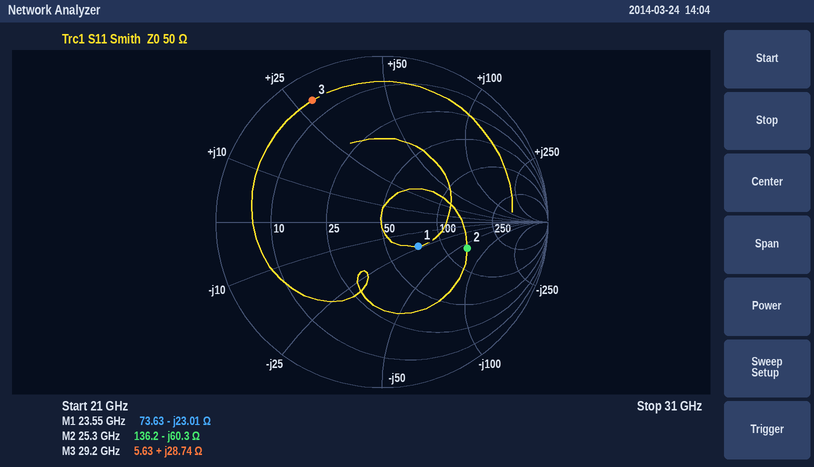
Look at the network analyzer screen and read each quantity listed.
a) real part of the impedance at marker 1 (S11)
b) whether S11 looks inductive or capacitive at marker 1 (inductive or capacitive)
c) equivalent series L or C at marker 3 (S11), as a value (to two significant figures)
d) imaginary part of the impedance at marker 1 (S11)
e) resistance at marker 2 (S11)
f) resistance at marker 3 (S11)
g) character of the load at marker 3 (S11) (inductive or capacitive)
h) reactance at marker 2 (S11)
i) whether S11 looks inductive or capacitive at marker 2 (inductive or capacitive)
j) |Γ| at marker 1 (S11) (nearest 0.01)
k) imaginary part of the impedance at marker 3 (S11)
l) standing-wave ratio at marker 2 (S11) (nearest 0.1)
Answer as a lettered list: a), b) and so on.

a) 73.63 Ω
b) capacitive
c) 160 pH
d) -23.01 Ω
e) 136.2 Ω
f) 5.63 Ω
g) inductive
h) -60.3 Ω
i) capacitive
j) 0.26
k) +28.74 Ω
l) 3.3
